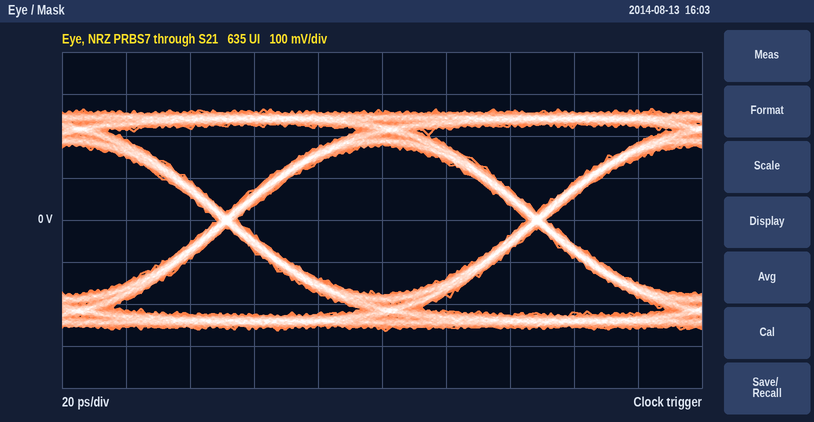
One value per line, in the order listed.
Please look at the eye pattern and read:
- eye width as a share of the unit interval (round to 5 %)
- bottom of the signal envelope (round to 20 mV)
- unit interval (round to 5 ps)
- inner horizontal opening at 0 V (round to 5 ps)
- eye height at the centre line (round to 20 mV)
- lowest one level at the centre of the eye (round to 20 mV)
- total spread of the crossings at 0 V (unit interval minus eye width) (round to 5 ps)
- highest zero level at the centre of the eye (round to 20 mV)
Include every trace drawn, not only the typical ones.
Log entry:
95 %
-260 mV
95 ps
90 ps
360 mV
180 mV
5 ps
-180 mV
